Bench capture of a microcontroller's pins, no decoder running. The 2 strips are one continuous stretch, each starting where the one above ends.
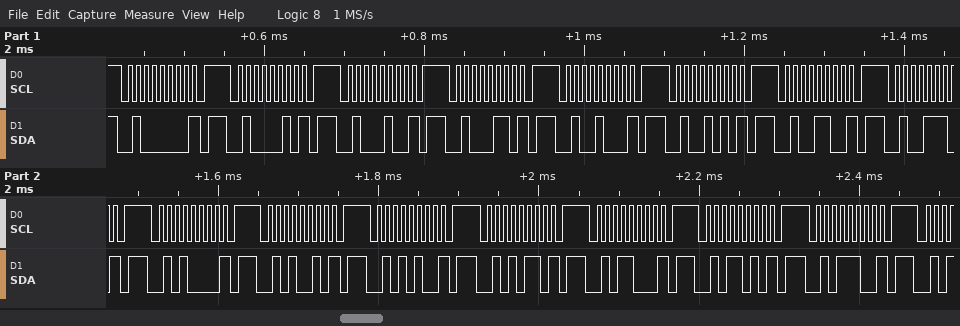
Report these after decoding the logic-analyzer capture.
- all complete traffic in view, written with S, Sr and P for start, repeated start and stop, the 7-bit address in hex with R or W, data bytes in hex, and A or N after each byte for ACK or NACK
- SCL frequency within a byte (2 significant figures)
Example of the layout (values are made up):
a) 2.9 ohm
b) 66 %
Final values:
a) S 20W N P S 21W N P S 22W N P S 23W N P S 24W N P S 25W N P S 26W N P S 27W N P S 28W N P S 29W N P S 2AW N P S 2BW N P S 2CW N P S 2DW N P S 2EW N P
b) 100 kHz
